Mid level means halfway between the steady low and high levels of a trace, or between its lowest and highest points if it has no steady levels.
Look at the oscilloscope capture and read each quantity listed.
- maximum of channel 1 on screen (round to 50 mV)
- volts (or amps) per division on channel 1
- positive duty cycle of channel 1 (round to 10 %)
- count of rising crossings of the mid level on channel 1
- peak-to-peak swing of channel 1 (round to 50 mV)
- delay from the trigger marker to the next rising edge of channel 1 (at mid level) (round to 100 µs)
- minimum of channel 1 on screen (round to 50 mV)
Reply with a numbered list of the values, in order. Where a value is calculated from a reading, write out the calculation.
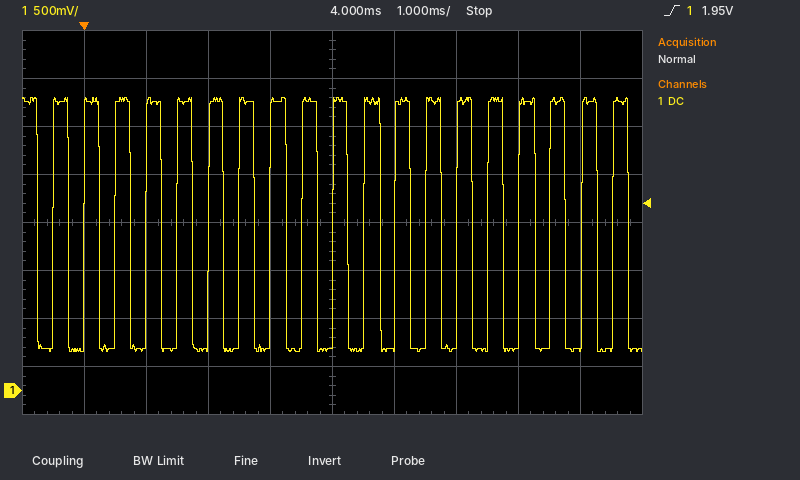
1. 3.05 V
2. 500 mV
3. 50 %
4. 19
5. 3.05 V − (400 mV) = 2.65 V
6. 500 µs
7. 400 mV
